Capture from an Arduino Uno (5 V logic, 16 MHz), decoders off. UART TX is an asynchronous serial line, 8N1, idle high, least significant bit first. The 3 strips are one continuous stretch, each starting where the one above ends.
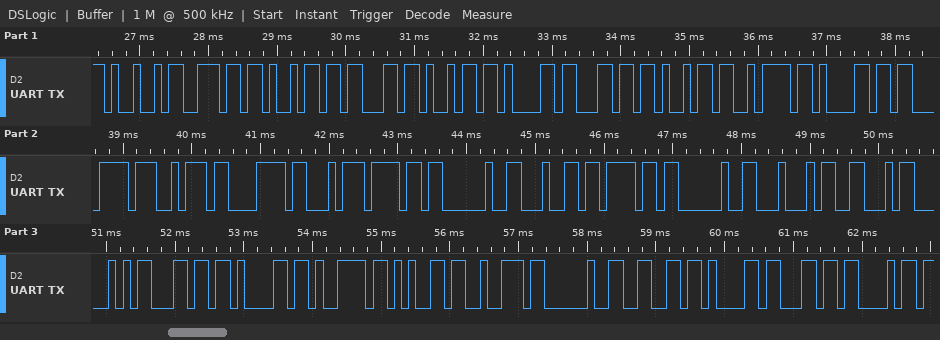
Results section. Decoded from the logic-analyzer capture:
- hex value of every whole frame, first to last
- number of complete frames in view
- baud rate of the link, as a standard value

49 6E 69 63 69 61 6C 69 7A 61 C3 A7 C3 A3 6F 20 64 6F 20 44 46 50 6C 61 79 65 72 20 66 61 6C 68
32
9600 baud
